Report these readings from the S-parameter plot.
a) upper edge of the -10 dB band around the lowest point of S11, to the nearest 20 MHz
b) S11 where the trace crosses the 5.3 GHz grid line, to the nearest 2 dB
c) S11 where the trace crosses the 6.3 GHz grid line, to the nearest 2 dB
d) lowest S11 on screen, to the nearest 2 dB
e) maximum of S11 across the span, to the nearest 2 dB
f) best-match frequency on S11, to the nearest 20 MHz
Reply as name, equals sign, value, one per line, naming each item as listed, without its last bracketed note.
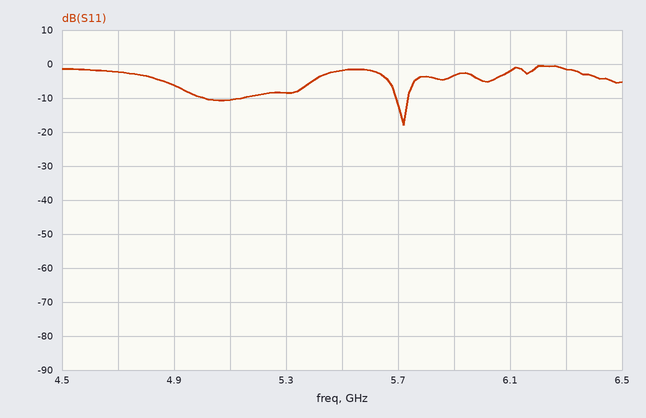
upper edge of the -10 dB band around the lowest point of S11, to the nearest 20 MHz = 5.74 GHz
S11 where the trace crosses the 5.3 GHz grid line, to the nearest 2 dB = -8 dB
S11 where the trace crosses the 6.3 GHz grid line, to the nearest 2 dB = -2 dB
lowest S11 on screen, to the nearest 2 dB = -18 dB
maximum of S11 across the span, to the nearest 2 dB = 0 dB
best-match frequency on S11, to the nearest 20 MHz = 5.72 GHz
